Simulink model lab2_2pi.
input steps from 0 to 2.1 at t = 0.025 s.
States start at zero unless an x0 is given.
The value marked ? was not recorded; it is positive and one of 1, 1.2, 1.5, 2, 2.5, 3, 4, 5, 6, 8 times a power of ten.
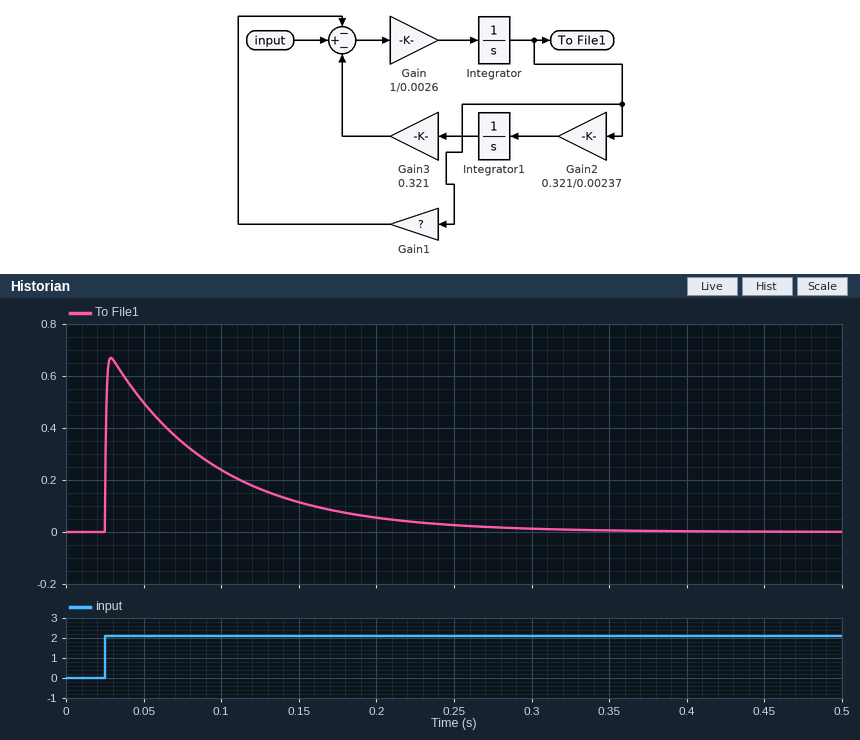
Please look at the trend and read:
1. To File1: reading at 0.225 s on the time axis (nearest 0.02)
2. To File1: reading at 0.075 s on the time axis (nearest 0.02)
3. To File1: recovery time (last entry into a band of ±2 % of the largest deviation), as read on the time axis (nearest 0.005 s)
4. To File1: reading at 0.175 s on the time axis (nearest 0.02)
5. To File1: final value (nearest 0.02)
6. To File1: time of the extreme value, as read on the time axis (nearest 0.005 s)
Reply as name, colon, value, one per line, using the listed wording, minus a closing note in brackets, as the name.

To File1: reading at 0.225 s on the time axis: 0.04
To File1: reading at 0.075 s on the time axis: 0.34
To File1: recovery time (last entry into a band of ±2 % of the largest deviation), as read on the time axis: 0.295 s
To File1: reading at 0.175 s on the time axis: 0.08
To File1: final value: 0.00
To File1: time of the extreme value, as read on the time axis: 0.030 s
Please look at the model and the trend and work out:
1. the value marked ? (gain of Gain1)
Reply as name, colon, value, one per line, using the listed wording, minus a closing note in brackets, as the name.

the value marked ?: 3
